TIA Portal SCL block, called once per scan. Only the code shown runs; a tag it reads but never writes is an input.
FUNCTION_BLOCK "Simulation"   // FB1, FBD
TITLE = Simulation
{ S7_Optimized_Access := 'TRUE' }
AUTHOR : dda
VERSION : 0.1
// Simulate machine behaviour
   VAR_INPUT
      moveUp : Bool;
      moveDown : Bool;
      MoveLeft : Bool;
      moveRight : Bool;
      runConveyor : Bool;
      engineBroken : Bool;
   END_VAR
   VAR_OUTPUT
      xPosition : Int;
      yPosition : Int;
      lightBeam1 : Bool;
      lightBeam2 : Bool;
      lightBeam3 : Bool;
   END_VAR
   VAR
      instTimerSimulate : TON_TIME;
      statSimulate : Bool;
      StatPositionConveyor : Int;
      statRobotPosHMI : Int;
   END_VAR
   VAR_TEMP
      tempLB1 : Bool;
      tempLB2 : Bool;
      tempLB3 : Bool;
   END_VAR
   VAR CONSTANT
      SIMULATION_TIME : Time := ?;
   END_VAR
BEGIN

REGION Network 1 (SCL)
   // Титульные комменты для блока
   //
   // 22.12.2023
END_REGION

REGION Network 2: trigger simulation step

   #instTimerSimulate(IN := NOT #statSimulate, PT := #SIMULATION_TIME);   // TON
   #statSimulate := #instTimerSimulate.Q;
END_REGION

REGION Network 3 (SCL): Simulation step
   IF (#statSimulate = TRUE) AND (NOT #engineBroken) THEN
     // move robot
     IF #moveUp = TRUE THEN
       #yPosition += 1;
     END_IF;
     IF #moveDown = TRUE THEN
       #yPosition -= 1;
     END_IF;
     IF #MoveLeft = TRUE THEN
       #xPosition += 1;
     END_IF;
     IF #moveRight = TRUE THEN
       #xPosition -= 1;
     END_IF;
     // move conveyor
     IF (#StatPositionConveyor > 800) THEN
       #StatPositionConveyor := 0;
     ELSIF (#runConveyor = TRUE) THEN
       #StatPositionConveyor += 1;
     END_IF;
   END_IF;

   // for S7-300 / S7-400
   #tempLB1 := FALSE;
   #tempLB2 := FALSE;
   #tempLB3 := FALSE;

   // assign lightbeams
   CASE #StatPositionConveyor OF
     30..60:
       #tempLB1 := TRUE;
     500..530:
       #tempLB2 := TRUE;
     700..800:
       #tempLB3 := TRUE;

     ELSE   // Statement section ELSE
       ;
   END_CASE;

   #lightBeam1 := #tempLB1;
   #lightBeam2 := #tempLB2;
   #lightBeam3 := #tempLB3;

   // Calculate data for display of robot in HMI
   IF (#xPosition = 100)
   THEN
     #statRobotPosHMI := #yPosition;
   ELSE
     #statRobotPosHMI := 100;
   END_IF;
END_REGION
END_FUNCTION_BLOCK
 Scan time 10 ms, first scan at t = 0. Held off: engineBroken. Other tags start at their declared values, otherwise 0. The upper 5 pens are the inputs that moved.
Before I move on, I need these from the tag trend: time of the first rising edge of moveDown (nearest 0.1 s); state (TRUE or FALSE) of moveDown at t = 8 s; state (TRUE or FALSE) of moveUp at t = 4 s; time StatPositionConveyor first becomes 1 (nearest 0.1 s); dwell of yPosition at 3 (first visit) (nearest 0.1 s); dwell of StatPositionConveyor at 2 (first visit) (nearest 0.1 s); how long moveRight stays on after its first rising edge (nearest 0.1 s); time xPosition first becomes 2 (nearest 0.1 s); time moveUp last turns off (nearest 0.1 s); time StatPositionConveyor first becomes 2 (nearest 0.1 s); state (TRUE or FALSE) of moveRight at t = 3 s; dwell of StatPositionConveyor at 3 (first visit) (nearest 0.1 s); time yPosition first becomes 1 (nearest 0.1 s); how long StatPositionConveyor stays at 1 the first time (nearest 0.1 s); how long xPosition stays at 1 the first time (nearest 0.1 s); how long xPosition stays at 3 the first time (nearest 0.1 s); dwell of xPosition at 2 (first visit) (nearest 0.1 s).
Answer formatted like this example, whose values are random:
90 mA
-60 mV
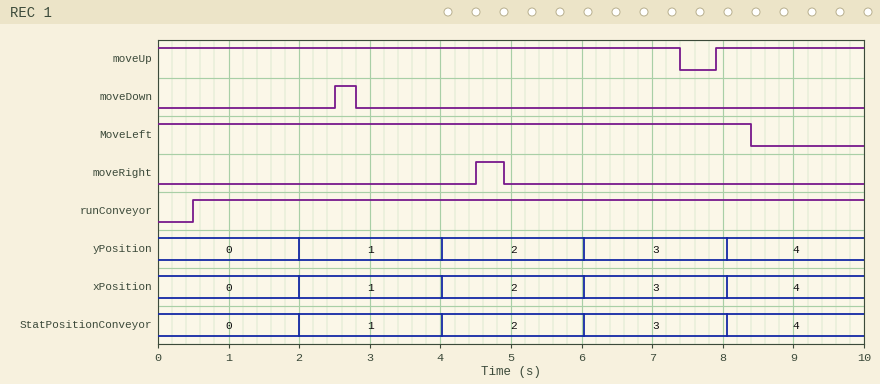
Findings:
2.5 s
FALSE
TRUE
2.0 s
2.0 s
2.0 s
0.4 s
4.0 s
7.4 s
4.0 s
FALSE
2.0 s
2.0 s
2.0 s
2.0 s
2.0 s
2.0 s
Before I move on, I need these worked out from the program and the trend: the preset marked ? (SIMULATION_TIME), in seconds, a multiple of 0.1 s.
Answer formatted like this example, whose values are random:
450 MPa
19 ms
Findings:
2.0 s
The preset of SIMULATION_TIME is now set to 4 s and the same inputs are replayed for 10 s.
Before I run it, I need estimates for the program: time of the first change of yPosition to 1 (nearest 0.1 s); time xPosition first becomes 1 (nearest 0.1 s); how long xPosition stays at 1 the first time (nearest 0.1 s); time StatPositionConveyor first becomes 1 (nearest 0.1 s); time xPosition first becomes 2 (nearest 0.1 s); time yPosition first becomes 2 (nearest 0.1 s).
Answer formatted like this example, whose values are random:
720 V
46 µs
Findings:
4.0 s
4.0 s
4.0 s
4.0 s
8.0 s
8.0 s
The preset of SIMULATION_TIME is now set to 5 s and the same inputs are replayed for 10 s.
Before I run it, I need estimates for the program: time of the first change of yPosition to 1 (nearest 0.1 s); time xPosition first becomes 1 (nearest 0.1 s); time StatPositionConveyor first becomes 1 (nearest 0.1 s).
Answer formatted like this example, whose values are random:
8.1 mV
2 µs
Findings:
5.0 s
5.0 s
5.0 s
